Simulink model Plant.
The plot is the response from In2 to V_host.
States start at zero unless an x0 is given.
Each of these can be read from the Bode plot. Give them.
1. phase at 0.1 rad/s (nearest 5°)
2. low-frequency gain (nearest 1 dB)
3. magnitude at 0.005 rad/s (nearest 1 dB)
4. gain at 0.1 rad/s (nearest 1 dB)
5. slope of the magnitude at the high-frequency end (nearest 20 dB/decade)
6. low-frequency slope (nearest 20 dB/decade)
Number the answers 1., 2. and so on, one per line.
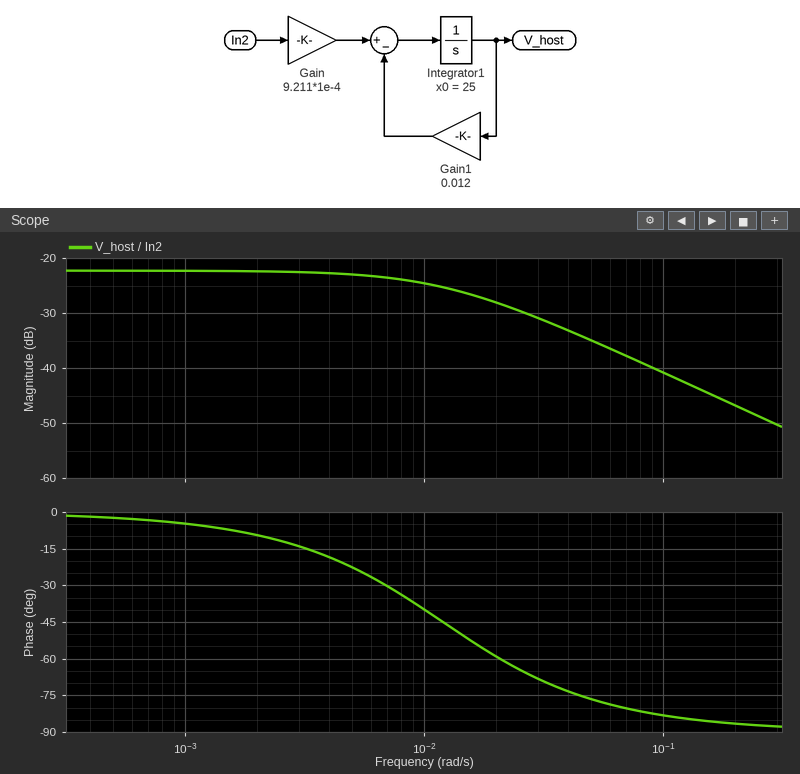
1. -85°
2. -22 dB
3. -23 dB
4. -41 dB
5. -20 dB/decade
6. 0 dB/decade
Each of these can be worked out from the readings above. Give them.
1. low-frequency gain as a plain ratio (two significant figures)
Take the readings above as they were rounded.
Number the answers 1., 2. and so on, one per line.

1. 0.079
